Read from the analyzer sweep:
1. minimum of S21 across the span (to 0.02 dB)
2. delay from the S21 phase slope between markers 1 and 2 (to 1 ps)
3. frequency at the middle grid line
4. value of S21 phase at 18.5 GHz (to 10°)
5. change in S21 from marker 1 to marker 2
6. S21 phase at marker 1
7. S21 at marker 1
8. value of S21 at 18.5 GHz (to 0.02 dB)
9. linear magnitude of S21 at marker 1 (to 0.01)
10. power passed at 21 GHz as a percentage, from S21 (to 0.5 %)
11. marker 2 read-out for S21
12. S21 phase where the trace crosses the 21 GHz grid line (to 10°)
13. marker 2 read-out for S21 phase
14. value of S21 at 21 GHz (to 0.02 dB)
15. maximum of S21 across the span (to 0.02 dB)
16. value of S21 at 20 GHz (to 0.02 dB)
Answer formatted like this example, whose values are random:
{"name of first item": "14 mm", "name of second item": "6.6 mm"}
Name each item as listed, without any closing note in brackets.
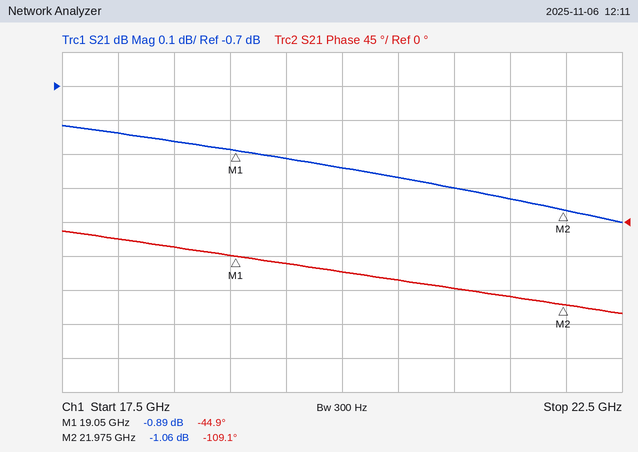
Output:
{"minimum of S21 across the span": "-1.10 dB", "delay from the S21 phase slope between markers 1 and 2": "61 ps", "frequency at the middle grid line": "20 GHz", "value of S21 phase at 18.5 GHz": "-30°", "change in S21 from marker 1 to marker 2": "-0.17 dB", "S21 phase at marker 1": "-44.9°", "S21 at marker 1": "-0.89 dB", "value of S21 at 18.5 GHz": "-0.86 dB", "linear magnitude of S21 at marker 1": "0.90", "power passed at 21 GHz as a percentage, from S21": "79.5 %", "marker 2 read-out for S21": "-1.06 dB", "S21 phase where the trace crosses the 21 GHz grid line": "-90°", "marker 2 read-out for S21 phase": "-109.1°", "value of S21 at 21 GHz": "-1.00 dB", "maximum of S21 across the span": "-0.82 dB", "value of S21 at 20 GHz": "-0.94 dB"}
